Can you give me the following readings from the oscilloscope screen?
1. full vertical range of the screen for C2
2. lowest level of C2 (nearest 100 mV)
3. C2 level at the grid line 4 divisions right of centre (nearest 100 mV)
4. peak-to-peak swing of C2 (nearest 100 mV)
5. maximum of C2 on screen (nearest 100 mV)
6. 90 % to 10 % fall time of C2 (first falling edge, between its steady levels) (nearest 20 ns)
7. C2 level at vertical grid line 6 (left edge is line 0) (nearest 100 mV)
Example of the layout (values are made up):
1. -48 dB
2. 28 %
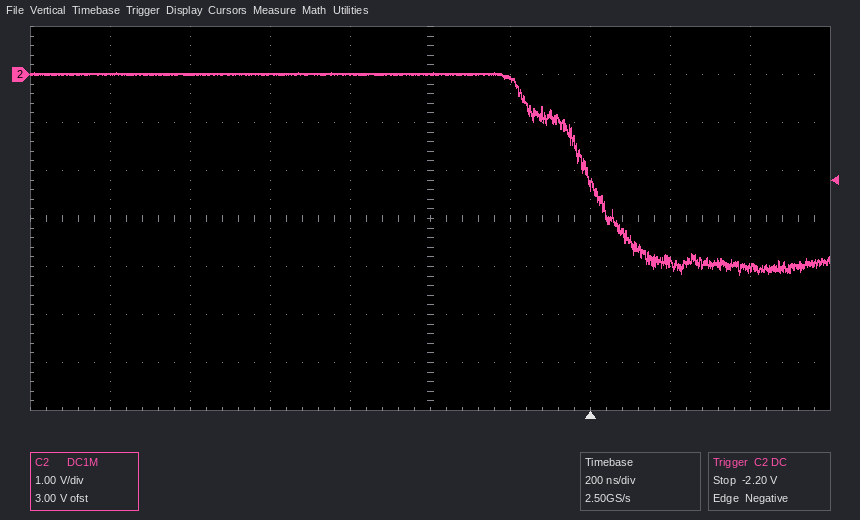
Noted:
1. 8 V
2. -4.2 V
3. -4.0 V
4. 4.2 V
5. 0.0 V
6. 280 ns
7. -100 mV
